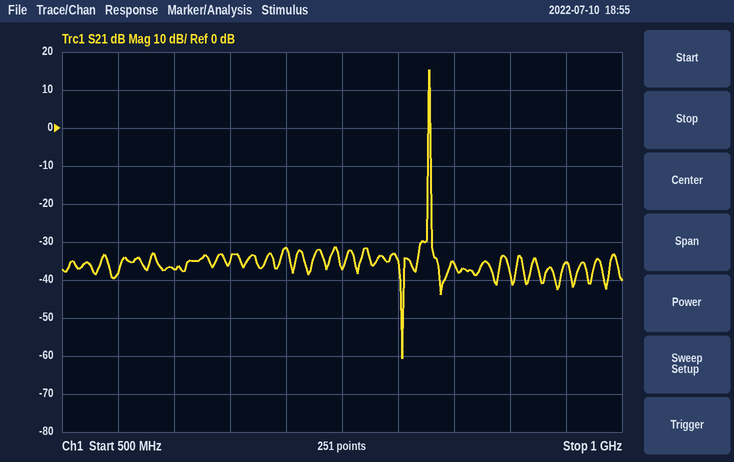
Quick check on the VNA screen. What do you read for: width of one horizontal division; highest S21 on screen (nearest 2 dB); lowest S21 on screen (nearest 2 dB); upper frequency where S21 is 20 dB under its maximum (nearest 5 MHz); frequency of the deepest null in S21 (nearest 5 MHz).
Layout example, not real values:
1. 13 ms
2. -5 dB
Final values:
1. 50 MHz
2. 16 dB
3. -60 dB
4. 830 MHz
5. 805 MHz
